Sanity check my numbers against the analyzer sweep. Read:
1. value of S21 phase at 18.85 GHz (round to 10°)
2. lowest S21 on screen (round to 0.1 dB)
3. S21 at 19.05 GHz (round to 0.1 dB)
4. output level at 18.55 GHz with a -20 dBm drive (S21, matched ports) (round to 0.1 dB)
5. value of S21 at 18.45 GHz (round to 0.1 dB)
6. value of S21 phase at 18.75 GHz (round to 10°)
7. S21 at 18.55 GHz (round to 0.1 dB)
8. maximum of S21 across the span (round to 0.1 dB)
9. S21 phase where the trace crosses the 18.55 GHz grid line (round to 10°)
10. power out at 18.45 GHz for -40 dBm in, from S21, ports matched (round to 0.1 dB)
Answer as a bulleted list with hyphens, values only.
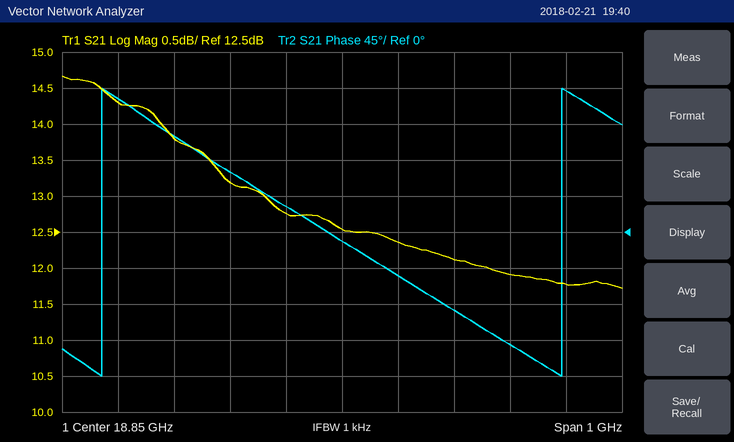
- -10°
- 11.7 dB
- 12.1 dB
- -6.2 dBm
- 14.3 dB
- 30°
- 13.8 dB
- 14.7 dB
- 120°
- -25.7 dBm
